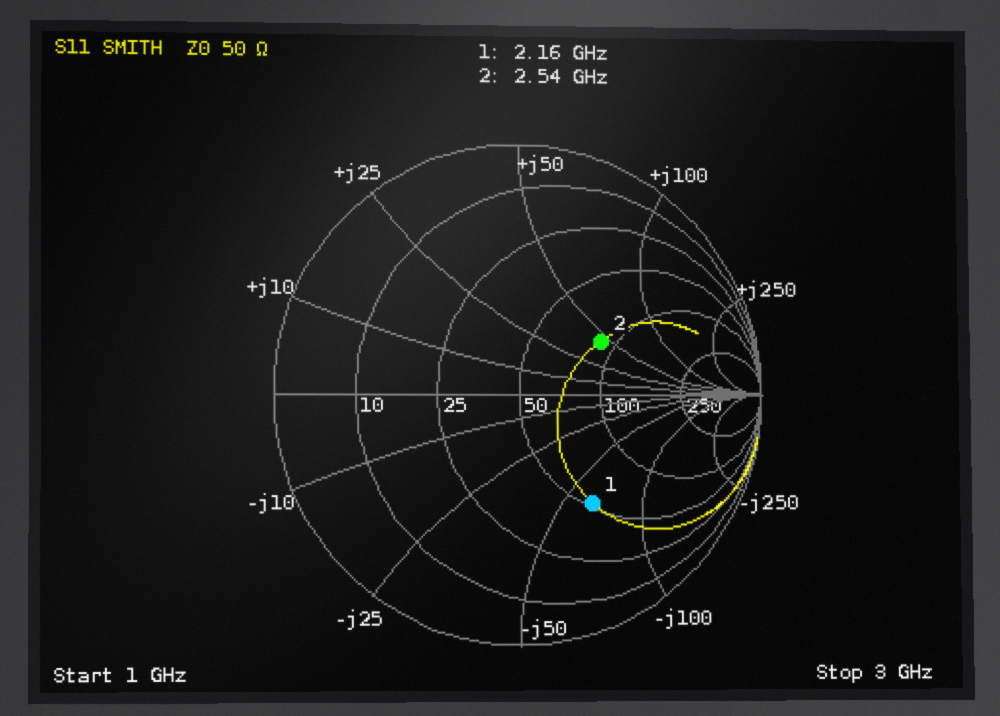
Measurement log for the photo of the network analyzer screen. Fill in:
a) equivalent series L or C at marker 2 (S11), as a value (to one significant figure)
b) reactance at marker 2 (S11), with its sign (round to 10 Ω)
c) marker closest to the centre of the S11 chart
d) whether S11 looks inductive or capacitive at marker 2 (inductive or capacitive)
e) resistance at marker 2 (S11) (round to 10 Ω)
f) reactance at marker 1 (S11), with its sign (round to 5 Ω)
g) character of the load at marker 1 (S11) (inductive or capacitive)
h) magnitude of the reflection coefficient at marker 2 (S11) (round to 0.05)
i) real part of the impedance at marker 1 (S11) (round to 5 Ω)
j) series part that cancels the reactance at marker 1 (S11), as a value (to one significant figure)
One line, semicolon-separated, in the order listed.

3 nH; +40 Ω; marker 2; inductive; 90 Ω; -65 Ω; capacitive; 0.40; 55 Ω; 5 nH
